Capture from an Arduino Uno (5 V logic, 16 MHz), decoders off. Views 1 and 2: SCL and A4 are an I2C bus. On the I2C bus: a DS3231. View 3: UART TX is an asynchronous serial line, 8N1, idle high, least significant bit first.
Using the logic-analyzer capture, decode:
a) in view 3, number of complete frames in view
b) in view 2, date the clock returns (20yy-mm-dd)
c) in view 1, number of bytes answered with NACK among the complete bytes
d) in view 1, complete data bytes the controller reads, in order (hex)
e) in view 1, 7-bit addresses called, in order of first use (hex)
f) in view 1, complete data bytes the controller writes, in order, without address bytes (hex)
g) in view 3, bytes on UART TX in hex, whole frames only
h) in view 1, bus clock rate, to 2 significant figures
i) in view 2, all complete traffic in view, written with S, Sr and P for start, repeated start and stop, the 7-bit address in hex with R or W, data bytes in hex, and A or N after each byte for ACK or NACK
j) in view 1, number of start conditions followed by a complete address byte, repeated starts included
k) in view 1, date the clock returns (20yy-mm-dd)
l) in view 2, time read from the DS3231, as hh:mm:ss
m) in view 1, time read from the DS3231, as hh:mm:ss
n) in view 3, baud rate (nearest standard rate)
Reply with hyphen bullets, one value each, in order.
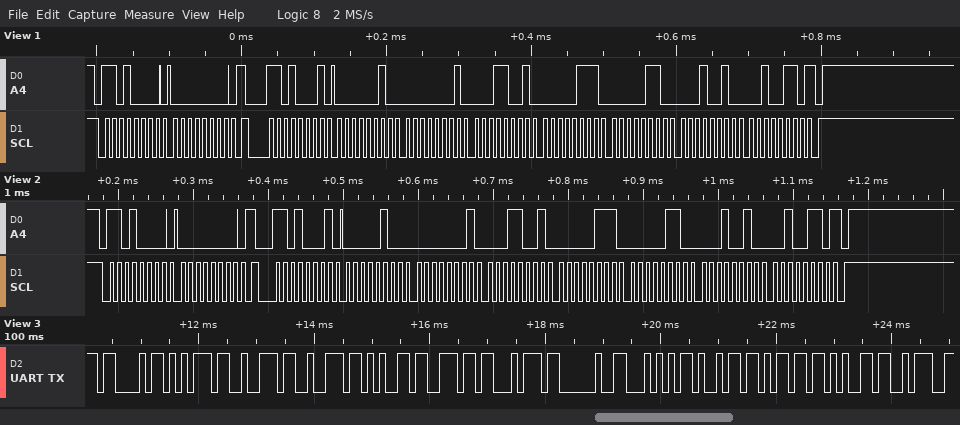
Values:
- 13
- 2026-12-06
- 1
- 02 01 19 07 06 12 26
- 0x68
- 00
- 43 75 72 72 65 6E 74 20 54 69 6D 65 3A
- 100 kHz
- S 68W A 00 A Sr 68R A 04 A 01 A 19 A 07 A 06 A 12 A 26 N P
- 2
- 2026-12-06
- 19:01:04
- 19:01:02
- 9600 baud
